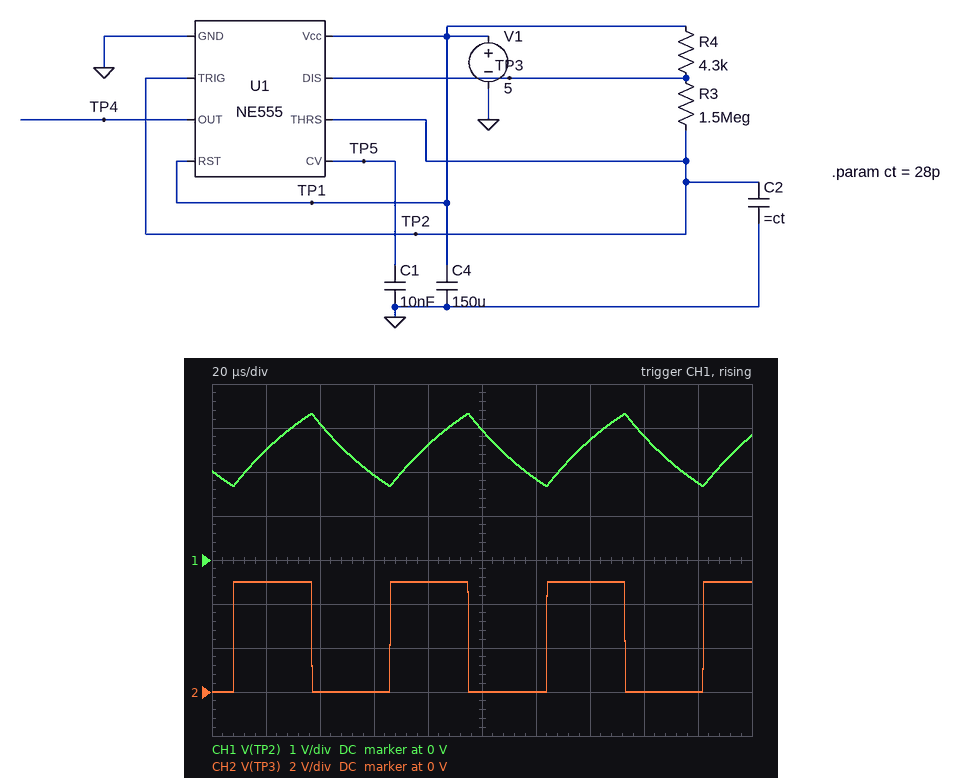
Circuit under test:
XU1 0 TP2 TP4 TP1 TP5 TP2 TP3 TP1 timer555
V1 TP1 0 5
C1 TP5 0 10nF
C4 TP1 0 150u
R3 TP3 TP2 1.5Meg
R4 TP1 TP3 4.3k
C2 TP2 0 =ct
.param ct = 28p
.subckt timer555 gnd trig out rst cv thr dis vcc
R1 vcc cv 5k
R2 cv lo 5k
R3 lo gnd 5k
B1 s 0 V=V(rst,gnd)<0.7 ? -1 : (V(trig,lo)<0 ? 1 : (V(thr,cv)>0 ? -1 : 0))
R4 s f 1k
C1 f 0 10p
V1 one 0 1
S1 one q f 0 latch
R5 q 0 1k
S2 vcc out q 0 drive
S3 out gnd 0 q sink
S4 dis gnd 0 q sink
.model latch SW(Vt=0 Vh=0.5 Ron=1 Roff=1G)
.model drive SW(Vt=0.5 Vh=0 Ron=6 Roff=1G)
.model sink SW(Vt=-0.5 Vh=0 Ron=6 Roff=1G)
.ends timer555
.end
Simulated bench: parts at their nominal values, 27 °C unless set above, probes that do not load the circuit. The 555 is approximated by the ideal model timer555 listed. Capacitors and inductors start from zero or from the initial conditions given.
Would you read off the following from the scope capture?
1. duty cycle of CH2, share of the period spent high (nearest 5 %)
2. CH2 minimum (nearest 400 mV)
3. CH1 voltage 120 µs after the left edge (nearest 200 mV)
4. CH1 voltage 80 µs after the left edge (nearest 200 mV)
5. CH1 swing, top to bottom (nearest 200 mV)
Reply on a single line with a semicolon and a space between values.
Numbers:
50 %; 0 V; 1.8 V; 2.6 V; 1.6 V
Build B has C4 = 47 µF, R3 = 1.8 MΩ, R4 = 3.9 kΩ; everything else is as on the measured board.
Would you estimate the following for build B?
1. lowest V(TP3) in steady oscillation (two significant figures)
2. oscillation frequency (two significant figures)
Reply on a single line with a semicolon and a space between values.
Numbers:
7.7 mV; 14 kHz
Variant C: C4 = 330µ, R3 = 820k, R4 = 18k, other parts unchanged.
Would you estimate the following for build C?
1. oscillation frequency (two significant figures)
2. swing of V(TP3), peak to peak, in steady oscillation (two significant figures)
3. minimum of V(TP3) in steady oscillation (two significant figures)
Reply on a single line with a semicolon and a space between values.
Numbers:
31 kHz; 5.0 V; 1.7 mV
